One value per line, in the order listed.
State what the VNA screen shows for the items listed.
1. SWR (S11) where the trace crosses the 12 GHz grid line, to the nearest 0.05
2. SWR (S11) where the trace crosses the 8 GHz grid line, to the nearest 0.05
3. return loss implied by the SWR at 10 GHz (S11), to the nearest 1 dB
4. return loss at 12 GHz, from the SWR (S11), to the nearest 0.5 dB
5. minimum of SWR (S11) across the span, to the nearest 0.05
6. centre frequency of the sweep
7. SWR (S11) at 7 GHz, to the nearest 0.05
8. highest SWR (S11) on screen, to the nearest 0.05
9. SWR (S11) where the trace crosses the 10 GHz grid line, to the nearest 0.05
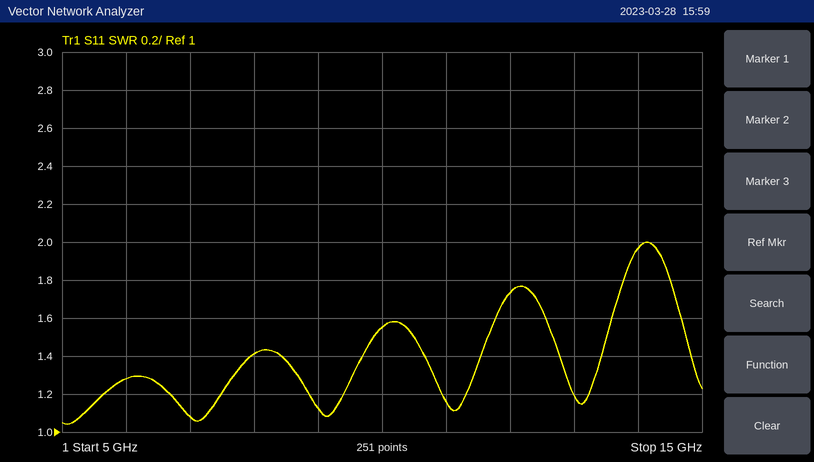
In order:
1.75
1.40
13 dB
11.5 dB
1.05
10 GHz
1.10
2.00
1.55
